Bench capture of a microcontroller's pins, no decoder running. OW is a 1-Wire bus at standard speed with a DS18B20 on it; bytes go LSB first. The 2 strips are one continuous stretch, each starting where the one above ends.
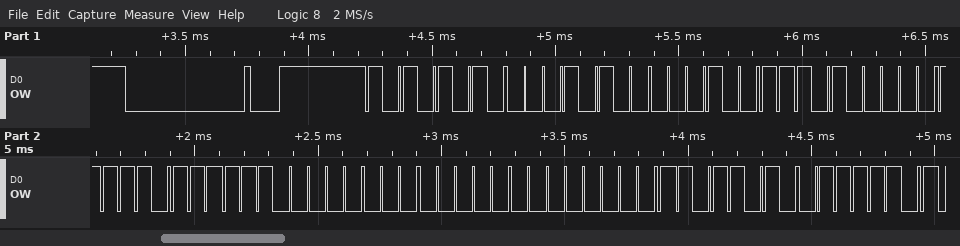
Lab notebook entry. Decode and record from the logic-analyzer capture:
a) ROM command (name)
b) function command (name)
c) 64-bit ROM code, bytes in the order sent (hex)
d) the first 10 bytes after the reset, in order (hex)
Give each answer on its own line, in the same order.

Match ROM
Read Scratchpad
28 C8 05 EF 07 00 00 5B
55 28 C8 05 EF 07 00 00 5B BE
